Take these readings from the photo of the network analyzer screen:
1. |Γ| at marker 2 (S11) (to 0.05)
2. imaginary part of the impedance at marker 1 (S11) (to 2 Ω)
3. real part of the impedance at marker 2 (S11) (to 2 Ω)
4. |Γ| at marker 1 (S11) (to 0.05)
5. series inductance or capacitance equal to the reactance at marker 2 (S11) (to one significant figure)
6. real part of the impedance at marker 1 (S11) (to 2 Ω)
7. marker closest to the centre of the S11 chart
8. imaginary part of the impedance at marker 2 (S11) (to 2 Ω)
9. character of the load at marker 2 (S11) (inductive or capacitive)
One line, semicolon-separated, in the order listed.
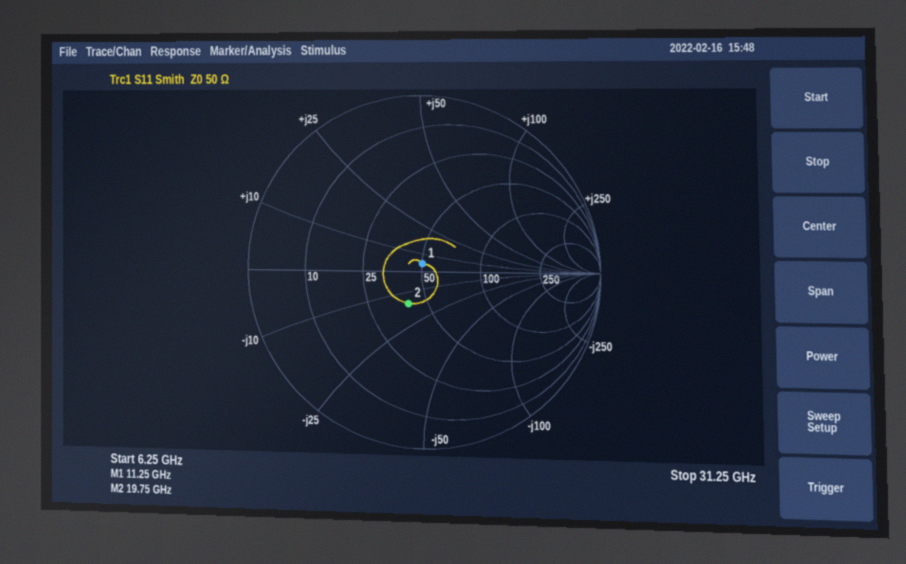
0.20; +4 Ω; 40 Ω; 0.05; 500 fF; 50 Ω; marker 1; -16 Ω; capacitive
